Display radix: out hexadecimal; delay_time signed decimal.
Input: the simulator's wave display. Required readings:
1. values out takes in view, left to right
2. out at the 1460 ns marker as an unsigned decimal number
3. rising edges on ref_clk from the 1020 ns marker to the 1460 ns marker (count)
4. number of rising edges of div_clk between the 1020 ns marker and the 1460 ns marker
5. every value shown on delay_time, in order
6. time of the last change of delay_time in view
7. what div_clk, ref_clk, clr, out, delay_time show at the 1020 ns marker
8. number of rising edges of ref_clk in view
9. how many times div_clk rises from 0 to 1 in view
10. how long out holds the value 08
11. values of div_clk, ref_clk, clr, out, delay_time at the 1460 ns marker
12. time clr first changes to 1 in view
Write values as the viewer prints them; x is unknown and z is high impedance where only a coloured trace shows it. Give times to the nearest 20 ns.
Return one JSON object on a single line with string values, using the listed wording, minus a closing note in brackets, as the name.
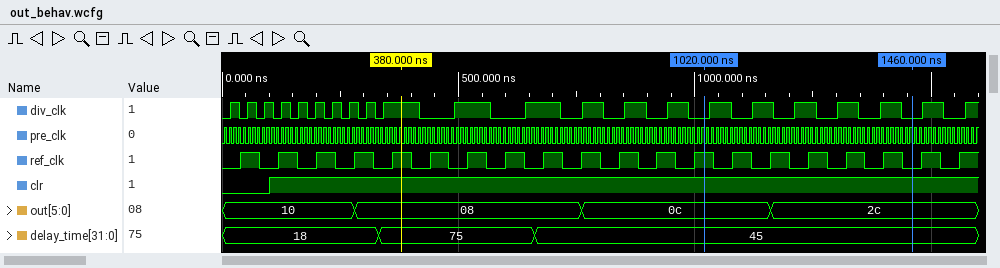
{"values out takes in view, left to right": "10, 08, 0c, 2c", "out at the 1460 ns marker as an unsigned decimal number": "44", "rising edges on ref_clk from the 1020 ns marker to the 1460 ns marker": "5", "number of rising edges of div_clk between the 1020 ns marker and the 1460 ns marker": "5", "every value shown on delay_time, in order": "18, 75, 45", "time of the last change of delay_time in view": "660 ns", "what div_clk, ref_clk, clr, out, delay_time show at the 1020 ns marker": "div_clk=0, ref_clk=1, clr=1, out=0c, delay_time=45", "number of rising edges of ref_clk in view": "20", "how many times div_clk rises from 0 to 1 in view": "22", "how long out holds the value 08": "480 ns", "values of div_clk, ref_clk, clr, out, delay_time at the 1460 ns marker": "div_clk=0, ref_clk=0, clr=1, out=2c, delay_time=45", "time clr first changes to 1 in view": "100 ns"}
